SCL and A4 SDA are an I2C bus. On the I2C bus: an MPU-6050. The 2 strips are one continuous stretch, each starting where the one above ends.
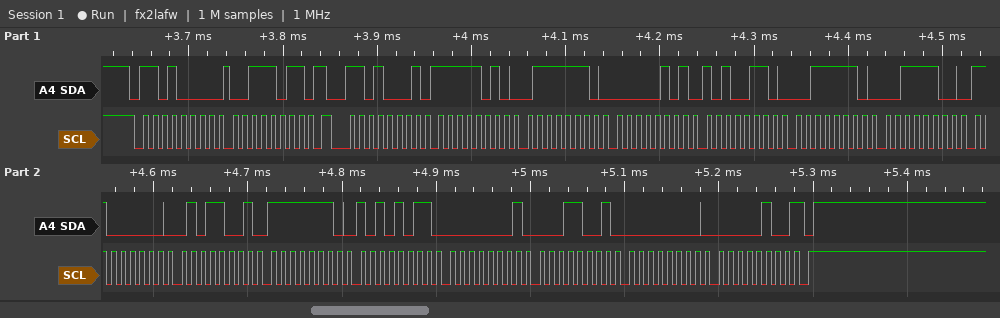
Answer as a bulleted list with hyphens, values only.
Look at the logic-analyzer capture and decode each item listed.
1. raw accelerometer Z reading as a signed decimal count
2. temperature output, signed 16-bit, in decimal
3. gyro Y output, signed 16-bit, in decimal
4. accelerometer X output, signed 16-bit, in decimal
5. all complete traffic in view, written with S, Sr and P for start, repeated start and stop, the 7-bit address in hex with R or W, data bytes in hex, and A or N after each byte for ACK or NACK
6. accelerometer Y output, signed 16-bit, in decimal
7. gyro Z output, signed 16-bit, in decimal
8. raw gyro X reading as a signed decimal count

- 15932
- -16295
- 281
- -1410
- S 68W A 3B A Sr 68R A FA A 7E A 05 A A6 A 3E A 3C A C0 A 59 A FE A AB A 01 A 19 A 00 A 04 N P
- 1446
- 4
- -341
